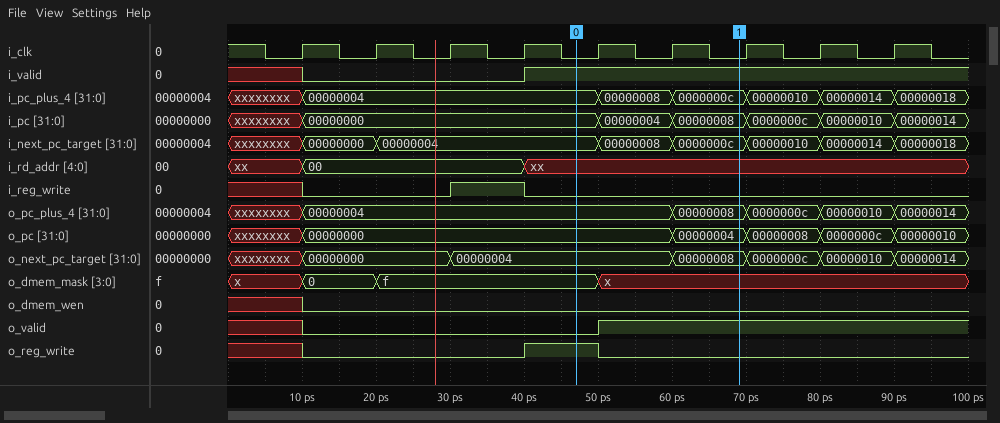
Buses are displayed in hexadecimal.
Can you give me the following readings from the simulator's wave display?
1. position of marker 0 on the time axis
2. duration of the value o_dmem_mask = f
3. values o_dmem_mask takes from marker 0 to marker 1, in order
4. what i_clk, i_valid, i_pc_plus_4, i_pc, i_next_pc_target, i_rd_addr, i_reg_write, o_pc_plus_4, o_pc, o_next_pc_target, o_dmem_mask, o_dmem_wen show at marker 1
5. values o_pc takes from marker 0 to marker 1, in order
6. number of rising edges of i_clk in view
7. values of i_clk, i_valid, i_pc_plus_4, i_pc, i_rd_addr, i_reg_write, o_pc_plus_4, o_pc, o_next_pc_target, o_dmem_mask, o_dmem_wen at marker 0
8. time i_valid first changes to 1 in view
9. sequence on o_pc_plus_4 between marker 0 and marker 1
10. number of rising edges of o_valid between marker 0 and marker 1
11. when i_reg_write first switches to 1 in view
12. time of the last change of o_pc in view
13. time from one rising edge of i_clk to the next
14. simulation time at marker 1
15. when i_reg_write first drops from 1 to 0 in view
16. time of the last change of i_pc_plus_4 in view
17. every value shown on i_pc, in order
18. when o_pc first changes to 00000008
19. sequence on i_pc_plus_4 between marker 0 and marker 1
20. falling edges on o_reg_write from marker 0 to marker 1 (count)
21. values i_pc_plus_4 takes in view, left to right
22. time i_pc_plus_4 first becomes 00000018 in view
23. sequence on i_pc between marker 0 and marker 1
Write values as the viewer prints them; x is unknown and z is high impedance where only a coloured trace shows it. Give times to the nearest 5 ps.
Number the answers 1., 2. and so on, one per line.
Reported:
1. 45 ps
2. 30 ps
3. f, x
4. i_clk=0, i_valid=1, i_pc_plus_4=0000000c, i_pc=00000008, i_next_pc_target=0000000c, i_rd_addr=xx, i_reg_write=0, o_pc_plus_4=00000008, o_pc=00000004, o_next_pc_target=00000008, o_dmem_mask=x, o_dmem_wen=0
5. 00000000, 00000004
6. 9
7. i_clk=0, i_valid=1, i_pc_plus_4=00000004, i_pc=00000000, i_rd_addr=xx, i_reg_write=0, o_pc_plus_4=00000004, o_pc=00000000, o_next_pc_target=00000004, o_dmem_mask=f, o_dmem_wen=0
8. 40 ps
9. 00000004, 00000008
10. 1
11. 30 ps
12. 90 ps
13. 10 ps
14. 70 ps
15. 40 ps
16. 90 ps
17. xxxxxxxx, 00000000, 00000004, 00000008, 0000000c, 00000010, 00000014
18. 70 ps
19. 00000004, 00000008, 0000000c
20. 1
21. xxxxxxxx, 00000004, 00000008, 0000000c, 00000010, 00000014, 00000018
22. 90 ps
23. 00000000, 00000004, 00000008
